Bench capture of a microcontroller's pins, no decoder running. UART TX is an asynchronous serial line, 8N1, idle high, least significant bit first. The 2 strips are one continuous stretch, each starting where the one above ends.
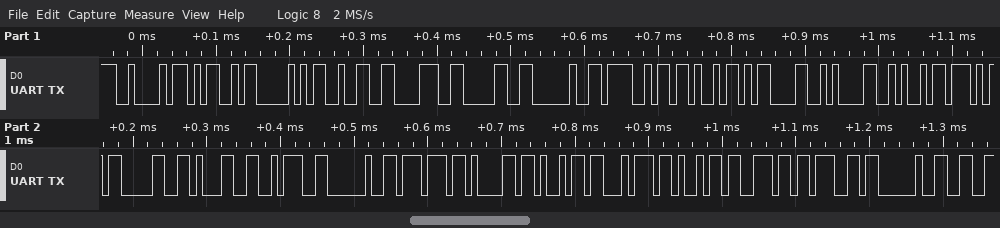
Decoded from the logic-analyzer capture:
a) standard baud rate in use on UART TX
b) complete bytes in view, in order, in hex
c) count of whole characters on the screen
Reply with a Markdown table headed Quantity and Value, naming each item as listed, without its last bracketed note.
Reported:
| Quantity | Value |
|---|---|
| standard baud rate in use on UART TX | 115200 baud |
| complete bytes in view, in order, in hex | 42 4D 50 32 38 30 20 4F 4B 0D 0A 4A 57 30 31 3A 20 77 61 69 74 69 6E 67 20 |
| count of whole characters on the screen | 25 |
